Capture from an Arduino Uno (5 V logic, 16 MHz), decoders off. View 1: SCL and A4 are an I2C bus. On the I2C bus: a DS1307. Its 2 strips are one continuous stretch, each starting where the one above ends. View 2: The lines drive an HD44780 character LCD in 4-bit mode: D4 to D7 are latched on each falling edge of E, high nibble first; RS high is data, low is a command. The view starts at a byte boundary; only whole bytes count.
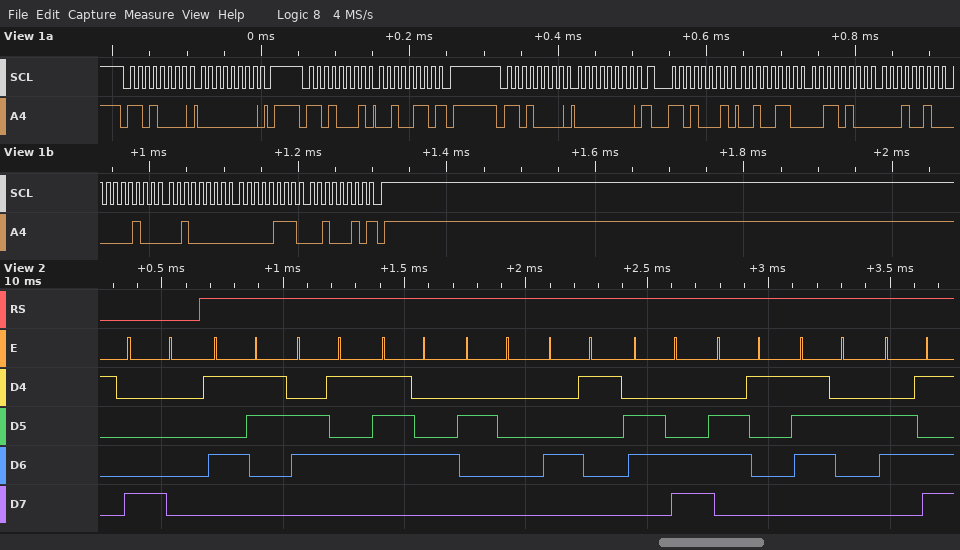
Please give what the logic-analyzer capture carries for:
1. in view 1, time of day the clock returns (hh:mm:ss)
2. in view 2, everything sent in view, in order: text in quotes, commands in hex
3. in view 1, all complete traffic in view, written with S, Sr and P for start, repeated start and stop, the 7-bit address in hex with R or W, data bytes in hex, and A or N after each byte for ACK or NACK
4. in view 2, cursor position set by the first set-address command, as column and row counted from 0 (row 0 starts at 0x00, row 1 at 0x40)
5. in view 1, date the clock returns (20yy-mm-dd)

12:34:26
0x80 "Set Alarm"
S 68W A 00 A P S 68R A 26 N P S 68W A 00 A Sr 68R A 26 A 34 A 12 A 04 A 20 A 07 A 22 N P
column 0, row 0
2022-07-20
